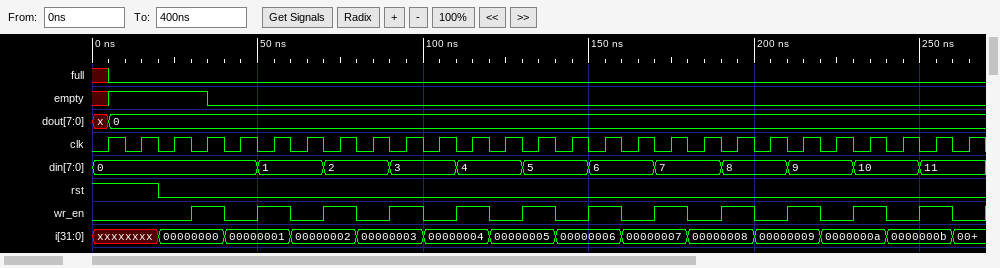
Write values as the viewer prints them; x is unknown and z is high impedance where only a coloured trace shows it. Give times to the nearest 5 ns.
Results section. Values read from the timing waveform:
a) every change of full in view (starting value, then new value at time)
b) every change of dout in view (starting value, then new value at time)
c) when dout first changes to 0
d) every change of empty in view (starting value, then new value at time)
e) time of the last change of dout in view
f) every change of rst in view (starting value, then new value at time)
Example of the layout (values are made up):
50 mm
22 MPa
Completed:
x, 0 at 5 ns
x, 0 at 5 ns
5 ns
x, 1 at 5 ns, 0 at 35 ns
5 ns
1, 0 at 20 ns
